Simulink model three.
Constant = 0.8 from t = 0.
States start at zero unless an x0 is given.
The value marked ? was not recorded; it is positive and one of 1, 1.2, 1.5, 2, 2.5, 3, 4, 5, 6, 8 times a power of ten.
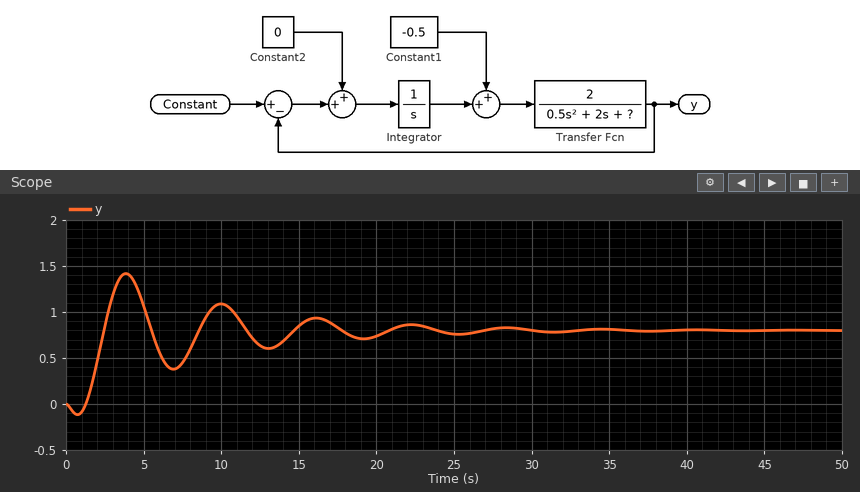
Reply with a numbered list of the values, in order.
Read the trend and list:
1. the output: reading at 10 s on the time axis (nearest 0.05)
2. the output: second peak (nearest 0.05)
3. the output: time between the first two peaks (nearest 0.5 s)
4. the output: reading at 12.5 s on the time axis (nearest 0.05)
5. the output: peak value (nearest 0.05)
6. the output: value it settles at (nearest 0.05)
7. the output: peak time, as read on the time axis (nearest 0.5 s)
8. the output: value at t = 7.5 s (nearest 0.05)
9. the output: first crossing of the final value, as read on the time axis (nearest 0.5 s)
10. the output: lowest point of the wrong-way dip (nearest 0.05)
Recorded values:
1. 1.10
2. 1.10
3. 6.0 s
4. 0.65
5. 1.40
6. 0.80
7. 4.0 s
8. 0.45
9. 2.5 s
10. -0.10
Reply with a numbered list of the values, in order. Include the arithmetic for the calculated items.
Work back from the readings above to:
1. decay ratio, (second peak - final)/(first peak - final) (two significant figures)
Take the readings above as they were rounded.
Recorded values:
1. (1.1 - 0.8) / (1.4 - 0.8) = 0.50
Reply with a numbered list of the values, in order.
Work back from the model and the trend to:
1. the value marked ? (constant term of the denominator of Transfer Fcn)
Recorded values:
1. 1
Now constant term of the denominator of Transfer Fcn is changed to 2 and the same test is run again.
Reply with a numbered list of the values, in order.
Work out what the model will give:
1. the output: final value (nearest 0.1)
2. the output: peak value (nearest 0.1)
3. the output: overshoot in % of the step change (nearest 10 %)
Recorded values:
1. 0.8
2. 1.0
3. 30 %
